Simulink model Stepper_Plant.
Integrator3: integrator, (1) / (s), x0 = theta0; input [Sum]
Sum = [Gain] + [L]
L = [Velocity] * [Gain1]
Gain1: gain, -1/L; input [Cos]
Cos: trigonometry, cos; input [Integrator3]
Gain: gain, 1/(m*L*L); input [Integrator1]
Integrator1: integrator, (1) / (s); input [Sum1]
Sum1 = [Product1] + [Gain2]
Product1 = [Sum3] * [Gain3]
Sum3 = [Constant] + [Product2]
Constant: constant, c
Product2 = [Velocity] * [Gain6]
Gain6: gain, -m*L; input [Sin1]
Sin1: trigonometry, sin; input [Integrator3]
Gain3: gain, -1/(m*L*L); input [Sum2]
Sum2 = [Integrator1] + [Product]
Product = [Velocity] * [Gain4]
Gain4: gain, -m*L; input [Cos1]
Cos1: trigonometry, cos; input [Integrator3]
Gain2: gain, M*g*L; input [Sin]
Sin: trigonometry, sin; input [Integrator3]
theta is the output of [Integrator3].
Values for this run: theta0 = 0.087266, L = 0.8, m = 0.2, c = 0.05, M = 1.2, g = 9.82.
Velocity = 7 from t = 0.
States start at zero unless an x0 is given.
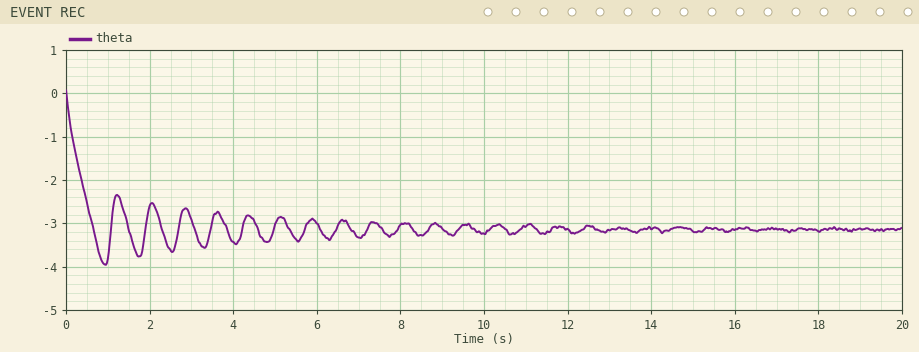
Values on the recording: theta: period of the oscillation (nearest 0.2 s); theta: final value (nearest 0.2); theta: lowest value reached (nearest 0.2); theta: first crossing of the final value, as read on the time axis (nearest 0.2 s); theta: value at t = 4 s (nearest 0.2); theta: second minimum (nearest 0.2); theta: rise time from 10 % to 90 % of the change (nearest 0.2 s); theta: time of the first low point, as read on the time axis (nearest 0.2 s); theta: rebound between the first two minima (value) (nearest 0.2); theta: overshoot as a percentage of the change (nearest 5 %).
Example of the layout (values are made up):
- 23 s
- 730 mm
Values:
- 0.8 s
- -3.2
- -4.0
- 0.6 s
- -3.4
- -3.8
- 0.6 s
- 1.0 s
- -2.4
- 25 %
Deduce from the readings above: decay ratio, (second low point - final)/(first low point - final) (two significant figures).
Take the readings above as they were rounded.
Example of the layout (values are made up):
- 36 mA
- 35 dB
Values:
- 0.75
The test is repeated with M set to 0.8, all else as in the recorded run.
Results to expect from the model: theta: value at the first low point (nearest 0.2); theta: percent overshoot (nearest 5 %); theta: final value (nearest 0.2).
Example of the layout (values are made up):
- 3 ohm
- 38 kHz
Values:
- -3.8
- 20 %
- -3.2
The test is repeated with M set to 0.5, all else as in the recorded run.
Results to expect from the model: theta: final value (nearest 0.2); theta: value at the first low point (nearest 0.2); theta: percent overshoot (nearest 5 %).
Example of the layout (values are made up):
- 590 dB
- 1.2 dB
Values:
- -3.2
- -3.6
- 15 %
